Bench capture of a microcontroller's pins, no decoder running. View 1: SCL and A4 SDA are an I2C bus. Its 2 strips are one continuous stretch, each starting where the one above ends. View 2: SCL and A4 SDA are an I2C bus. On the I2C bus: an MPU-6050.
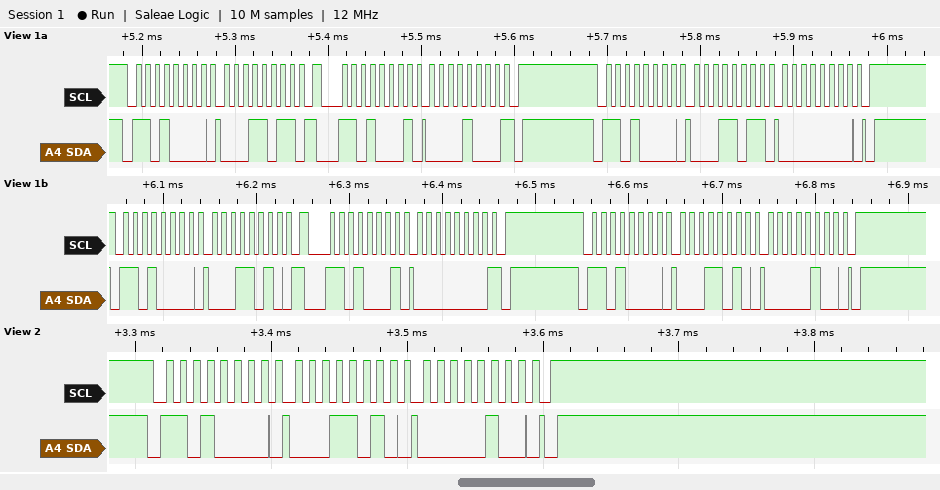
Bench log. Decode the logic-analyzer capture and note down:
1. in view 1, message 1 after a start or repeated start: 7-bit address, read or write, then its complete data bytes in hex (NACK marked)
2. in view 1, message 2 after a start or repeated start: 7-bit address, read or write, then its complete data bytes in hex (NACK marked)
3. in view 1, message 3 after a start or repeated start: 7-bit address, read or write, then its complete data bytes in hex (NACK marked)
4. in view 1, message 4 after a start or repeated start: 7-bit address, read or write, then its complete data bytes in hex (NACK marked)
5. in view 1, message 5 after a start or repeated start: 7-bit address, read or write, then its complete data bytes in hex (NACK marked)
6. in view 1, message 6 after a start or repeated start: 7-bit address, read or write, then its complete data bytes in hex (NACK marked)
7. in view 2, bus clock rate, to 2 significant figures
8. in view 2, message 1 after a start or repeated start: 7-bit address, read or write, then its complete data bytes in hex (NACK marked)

0x68 write: 1B
0x68 read: 08 NACK
0x68 write: 1B 00
0x68 write: 1A
0x68 read: 00 NACK
0x68 write: 1A 04
100 kHz
0x68 write: 1A 04
